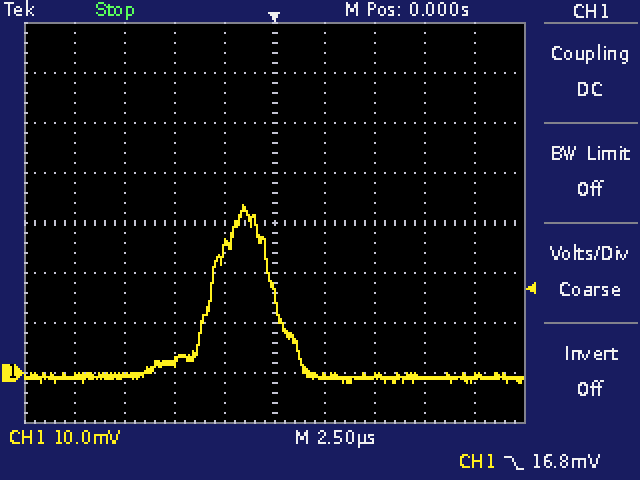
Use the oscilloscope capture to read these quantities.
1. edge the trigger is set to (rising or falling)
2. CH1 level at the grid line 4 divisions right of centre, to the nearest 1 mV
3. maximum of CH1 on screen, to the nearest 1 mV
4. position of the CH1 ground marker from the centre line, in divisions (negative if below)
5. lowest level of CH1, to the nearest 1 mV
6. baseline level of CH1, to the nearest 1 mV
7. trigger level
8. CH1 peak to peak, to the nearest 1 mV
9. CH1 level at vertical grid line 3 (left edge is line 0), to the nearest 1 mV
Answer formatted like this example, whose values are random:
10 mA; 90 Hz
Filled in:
falling; -1 mV; 34 mV; -3.0 div; -2 mV; -1 mV; 16.8 mV; 36 mV; 2 mV
